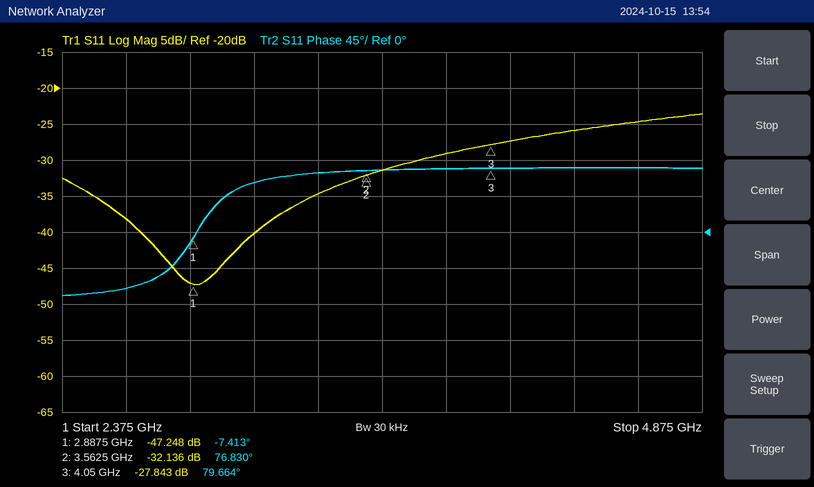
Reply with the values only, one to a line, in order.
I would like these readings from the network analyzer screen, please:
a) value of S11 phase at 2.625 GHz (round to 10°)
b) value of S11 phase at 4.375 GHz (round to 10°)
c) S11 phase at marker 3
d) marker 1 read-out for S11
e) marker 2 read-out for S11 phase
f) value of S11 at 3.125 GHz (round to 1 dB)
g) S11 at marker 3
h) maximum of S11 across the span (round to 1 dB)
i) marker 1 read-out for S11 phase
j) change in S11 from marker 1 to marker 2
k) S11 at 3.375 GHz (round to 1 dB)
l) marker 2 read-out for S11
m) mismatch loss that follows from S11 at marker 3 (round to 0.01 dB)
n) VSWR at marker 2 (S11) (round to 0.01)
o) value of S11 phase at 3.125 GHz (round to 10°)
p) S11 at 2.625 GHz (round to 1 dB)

-70°
80°
79.664°
-47.248 dB
76.830°
-40 dB
-27.843 dB
-24 dB
-7.413°
15.112 dB
-35 dB
-32.136 dB
0.01 dB
1.05
60°
-38 dB
